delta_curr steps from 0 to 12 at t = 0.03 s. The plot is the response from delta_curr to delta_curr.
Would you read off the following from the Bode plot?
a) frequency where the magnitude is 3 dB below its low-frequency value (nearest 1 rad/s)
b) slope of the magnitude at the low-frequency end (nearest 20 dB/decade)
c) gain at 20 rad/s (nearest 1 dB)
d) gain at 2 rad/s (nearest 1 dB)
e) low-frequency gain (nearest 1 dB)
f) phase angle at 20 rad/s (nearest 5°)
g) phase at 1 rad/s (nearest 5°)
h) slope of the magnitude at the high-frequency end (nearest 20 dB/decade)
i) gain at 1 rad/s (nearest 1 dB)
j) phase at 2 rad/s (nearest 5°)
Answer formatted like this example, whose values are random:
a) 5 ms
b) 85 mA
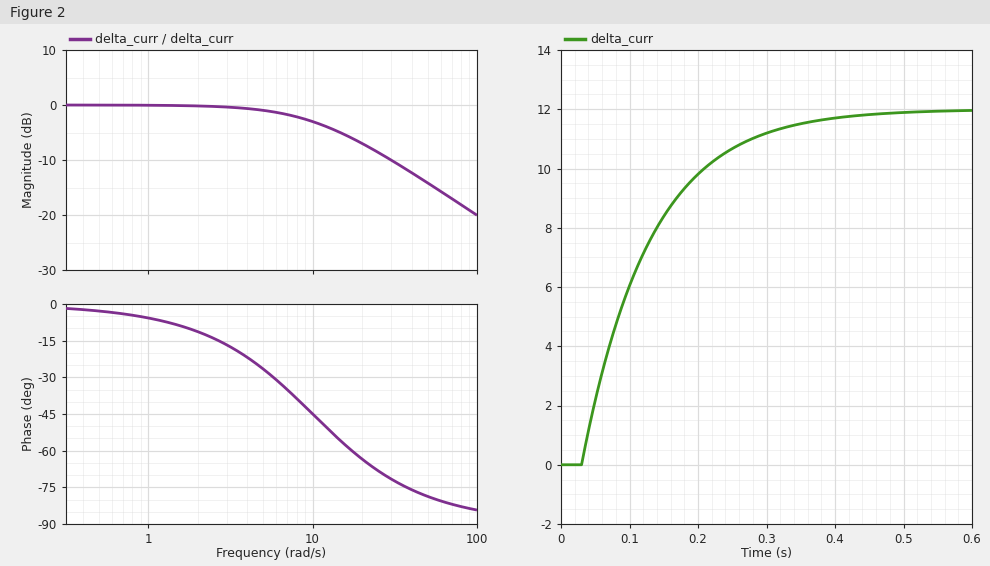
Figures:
a) 10 rad/s
b) 0 dB/decade
c) -7 dB
d) 0 dB
e) 0 dB
f) -65°
g) -5°
h) -20 dB/decade
i) 0 dB
j) -10°
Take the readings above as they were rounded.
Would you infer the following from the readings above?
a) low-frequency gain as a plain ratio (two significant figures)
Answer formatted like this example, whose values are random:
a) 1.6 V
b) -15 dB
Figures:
a) 1.0
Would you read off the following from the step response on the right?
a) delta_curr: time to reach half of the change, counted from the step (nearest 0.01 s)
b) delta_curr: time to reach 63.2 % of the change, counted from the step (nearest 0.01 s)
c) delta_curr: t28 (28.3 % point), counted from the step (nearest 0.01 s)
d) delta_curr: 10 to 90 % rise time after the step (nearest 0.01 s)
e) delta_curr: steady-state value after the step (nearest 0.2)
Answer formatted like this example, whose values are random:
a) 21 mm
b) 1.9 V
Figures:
a) 0.07 s
b) 0.10 s
c) 0.03 s
d) 0.22 s
e) 12.0
